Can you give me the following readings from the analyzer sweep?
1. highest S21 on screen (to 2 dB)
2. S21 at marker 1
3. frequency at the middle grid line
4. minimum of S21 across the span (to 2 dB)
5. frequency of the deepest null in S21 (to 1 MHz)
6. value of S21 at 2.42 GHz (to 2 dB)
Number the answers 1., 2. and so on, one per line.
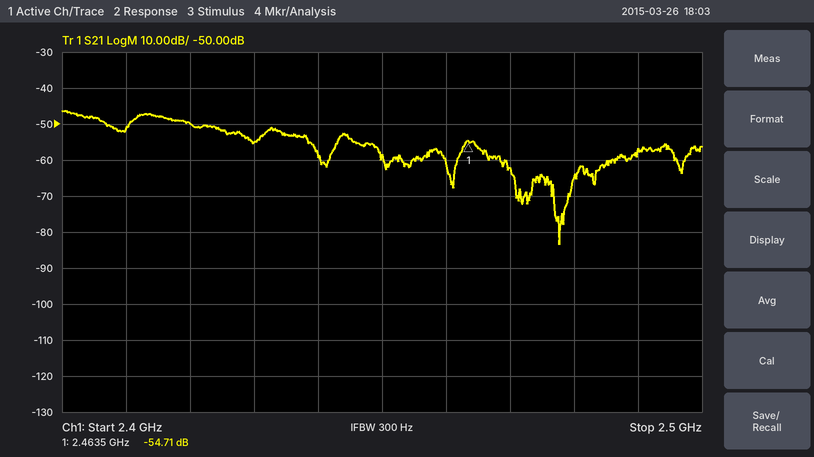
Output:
1. -46 dB
2. -54.71 dB
3. 2.45 GHz
4. -84 dB
5. 2.478 GHz
6. -50 dB
